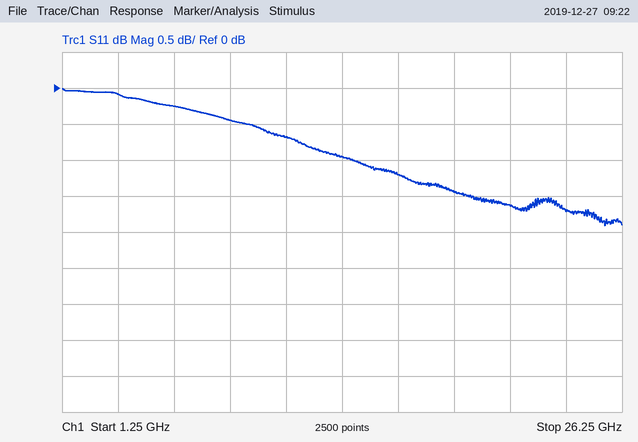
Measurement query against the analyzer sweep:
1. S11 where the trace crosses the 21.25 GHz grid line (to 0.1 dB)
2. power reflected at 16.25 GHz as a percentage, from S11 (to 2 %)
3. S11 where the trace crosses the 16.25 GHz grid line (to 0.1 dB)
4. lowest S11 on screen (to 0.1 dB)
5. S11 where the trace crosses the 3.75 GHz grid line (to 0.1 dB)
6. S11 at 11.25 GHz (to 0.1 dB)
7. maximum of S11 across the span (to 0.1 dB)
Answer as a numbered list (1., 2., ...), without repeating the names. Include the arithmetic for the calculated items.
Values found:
1. -1.6 dB
2. 10^(-1.2/10) ≈ 76 %
3. -1.2 dB
4. -1.9 dB
5. -0.1 dB
6. -0.7 dB
7. 0.0 dB
